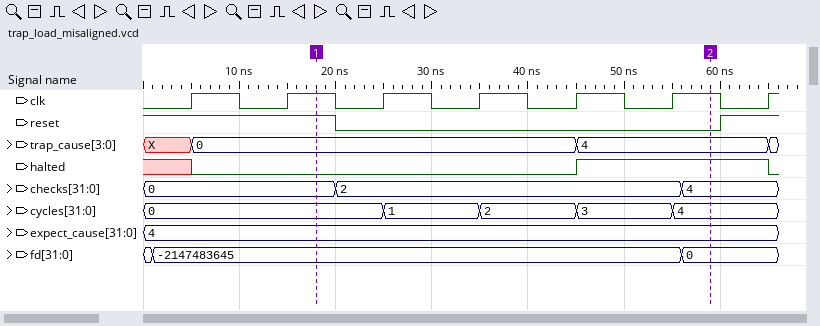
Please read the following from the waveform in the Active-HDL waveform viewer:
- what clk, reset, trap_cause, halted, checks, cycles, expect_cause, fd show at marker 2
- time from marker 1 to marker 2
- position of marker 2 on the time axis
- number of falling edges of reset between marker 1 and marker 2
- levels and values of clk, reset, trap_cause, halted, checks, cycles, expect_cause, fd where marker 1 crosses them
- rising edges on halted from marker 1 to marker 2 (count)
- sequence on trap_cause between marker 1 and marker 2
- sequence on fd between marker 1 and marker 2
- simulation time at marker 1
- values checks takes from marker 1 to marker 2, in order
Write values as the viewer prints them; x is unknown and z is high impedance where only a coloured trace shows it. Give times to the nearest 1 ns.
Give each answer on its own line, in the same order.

clk=1, reset=0, trap_cause=4, halted=1, checks=4, cycles=4, expect_cause=4, fd=0
41 ns
59 ns
1
clk=1, reset=1, trap_cause=0, halted=0, checks=0, cycles=0, expect_cause=4, fd=-2147483645
1
0, 4
-2147483645, 0
18 ns
0, 2, 4
